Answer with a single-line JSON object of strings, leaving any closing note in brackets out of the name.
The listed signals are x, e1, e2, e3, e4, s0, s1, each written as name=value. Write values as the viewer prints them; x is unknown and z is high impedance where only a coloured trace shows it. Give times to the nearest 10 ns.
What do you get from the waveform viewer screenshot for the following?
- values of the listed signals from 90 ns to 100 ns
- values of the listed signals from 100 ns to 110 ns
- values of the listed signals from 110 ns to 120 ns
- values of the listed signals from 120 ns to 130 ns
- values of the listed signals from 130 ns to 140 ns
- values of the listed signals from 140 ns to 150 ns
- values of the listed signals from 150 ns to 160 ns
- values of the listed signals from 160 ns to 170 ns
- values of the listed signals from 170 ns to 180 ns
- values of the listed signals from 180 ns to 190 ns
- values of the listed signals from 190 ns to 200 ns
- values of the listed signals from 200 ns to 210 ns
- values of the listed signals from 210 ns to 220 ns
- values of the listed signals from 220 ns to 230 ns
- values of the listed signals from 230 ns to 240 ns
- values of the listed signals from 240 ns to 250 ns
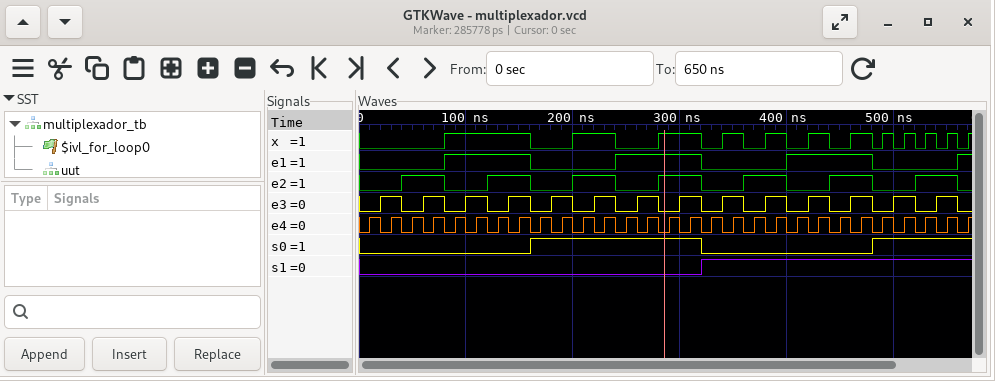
{"values of the listed signals from 90 ns to 100 ns": "x=1, e1=1, e2=0, e3=0, e4=1, s0=0, s1=0", "values of the listed signals from 100 ns to 110 ns": "x=1, e1=1, e2=0, e3=1, e4=0, s0=0, s1=0", "values of the listed signals from 110 ns to 120 ns": "x=1, e1=1, e2=0, e3=1, e4=1, s0=0, s1=0", "values of the listed signals from 120 ns to 130 ns": "x=1, e1=1, e2=1, e3=0, e4=0, s0=0, s1=0", "values of the listed signals from 130 ns to 140 ns": "x=1, e1=1, e2=1, e3=0, e4=1, s0=0, s1=0", "values of the listed signals from 140 ns to 150 ns": "x=1, e1=1, e2=1, e3=1, e4=0, s0=0, s1=0", "values of the listed signals from 150 ns to 160 ns": "x=1, e1=1, e2=1, e3=1, e4=1, s0=0, s1=0", "values of the listed signals from 160 ns to 170 ns": "x=0, e1=0, e2=0, e3=0, e4=0, s0=1, s1=0", "values of the listed signals from 170 ns to 180 ns": "x=0, e1=0, e2=0, e3=0, e4=1, s0=1, s1=0", "values of the listed signals from 180 ns to 190 ns": "x=0, e1=0, e2=0, e3=1, e4=0, s0=1, s1=0", "values of the listed signals from 190 ns to 200 ns": "x=0, e1=0, e2=0, e3=1, e4=1, s0=1, s1=0", "values of the listed signals from 200 ns to 210 ns": "x=1, e1=0, e2=1, e3=0, e4=0, s0=1, s1=0", "values of the listed signals from 210 ns to 220 ns": "x=1, e1=0, e2=1, e3=0, e4=1, s0=1, s1=0", "values of the listed signals from 220 ns to 230 ns": "x=1, e1=0, e2=1, e3=1, e4=0, s0=1, s1=0", "values of the listed signals from 230 ns to 240 ns": "x=1, e1=0, e2=1, e3=1, e4=1, s0=1, s1=0", "values of the listed signals from 240 ns to 250 ns": "x=0, e1=1, e2=0, e3=0, e4=0, s0=1, s1=0"}
